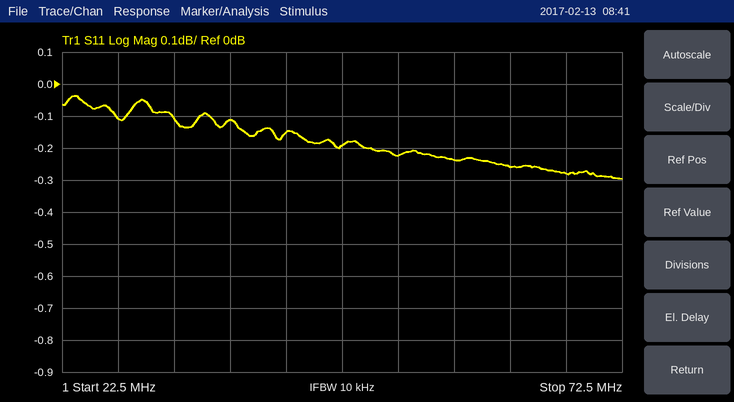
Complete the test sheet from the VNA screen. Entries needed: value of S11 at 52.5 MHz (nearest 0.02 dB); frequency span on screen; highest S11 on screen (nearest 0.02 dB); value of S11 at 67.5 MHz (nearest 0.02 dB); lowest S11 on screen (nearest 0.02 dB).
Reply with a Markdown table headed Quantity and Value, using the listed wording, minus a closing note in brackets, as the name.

| Quantity | Value |
|---|---|
| value of S11 at 52.5 MHz | -0.22 dB |
| frequency span on screen | 50 MHz |
| highest S11 on screen | -0.04 dB |
| value of S11 at 67.5 MHz | -0.28 dB |
| lowest S11 on screen | -0.30 dB |
